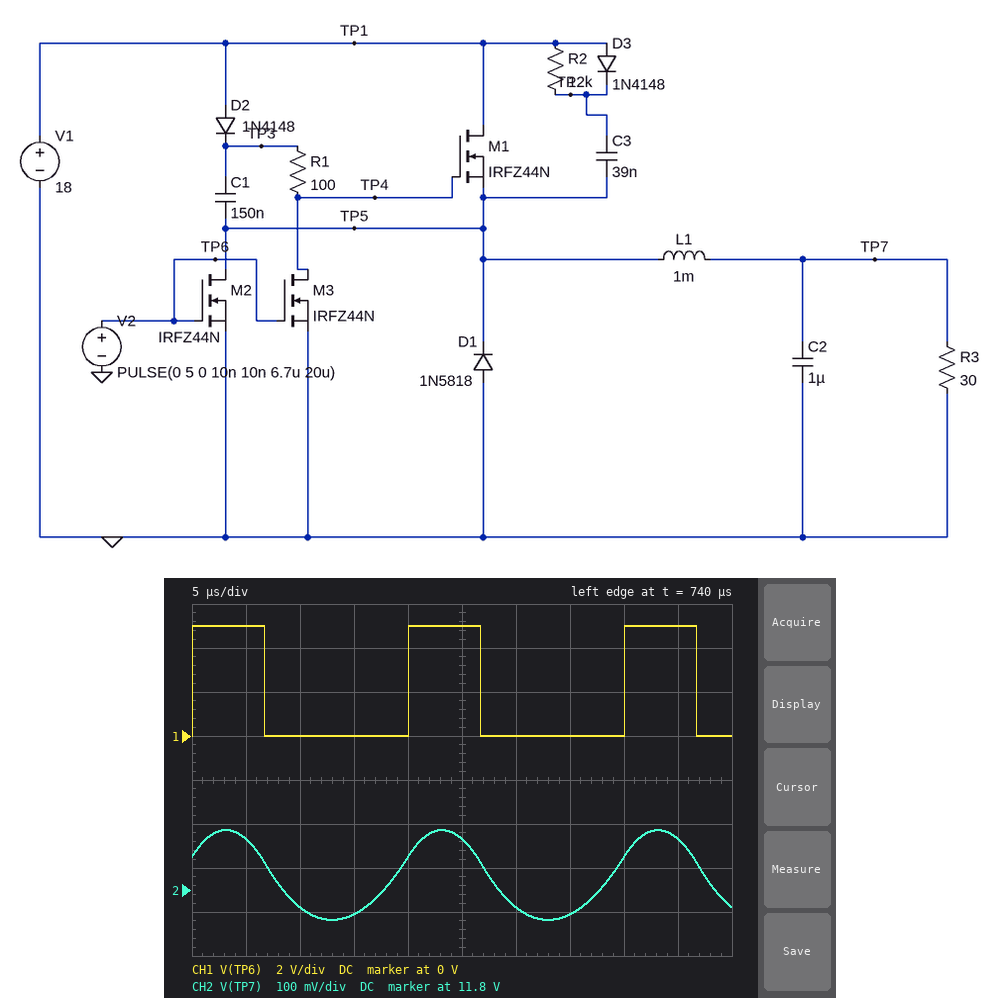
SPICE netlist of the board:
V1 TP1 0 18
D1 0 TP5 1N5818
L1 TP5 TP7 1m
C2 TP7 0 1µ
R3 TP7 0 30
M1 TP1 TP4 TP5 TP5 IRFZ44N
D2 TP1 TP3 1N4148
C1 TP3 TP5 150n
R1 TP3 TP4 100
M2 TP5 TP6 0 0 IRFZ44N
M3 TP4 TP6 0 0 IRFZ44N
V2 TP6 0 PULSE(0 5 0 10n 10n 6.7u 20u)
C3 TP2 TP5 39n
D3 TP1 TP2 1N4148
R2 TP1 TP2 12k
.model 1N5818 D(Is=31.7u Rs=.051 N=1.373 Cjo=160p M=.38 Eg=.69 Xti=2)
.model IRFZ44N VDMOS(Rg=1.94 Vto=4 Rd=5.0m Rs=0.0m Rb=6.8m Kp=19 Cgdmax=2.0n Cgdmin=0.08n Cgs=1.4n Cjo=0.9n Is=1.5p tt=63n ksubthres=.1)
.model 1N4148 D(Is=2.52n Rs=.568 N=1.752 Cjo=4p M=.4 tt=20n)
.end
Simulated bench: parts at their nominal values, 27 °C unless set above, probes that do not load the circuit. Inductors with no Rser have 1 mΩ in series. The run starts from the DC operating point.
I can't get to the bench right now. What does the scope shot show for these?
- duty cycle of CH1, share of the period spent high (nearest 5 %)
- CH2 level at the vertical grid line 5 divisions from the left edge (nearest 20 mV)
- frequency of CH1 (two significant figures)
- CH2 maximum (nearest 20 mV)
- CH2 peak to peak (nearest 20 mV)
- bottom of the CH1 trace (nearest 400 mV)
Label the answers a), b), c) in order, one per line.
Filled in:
a) 35 %
b) 11.92 V
c) 50 kHz
d) 11.94 V
e) 200 mV
f) 0 V
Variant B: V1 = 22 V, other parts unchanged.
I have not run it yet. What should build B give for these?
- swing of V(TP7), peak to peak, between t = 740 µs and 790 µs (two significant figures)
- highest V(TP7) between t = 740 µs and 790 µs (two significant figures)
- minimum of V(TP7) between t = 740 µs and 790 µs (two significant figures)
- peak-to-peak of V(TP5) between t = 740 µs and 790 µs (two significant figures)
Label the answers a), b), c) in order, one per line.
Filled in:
a) 250 mV
b) 15 V
c) 14 V
d) 22 V
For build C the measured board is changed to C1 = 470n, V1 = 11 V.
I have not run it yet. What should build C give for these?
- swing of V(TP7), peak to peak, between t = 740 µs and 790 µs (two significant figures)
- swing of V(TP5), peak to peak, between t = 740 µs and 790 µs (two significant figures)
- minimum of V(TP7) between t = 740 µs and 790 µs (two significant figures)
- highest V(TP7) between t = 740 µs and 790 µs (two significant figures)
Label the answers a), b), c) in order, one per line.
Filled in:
a) 130 mV
b) 11 V
c) 7.1 V
d) 7.2 V
